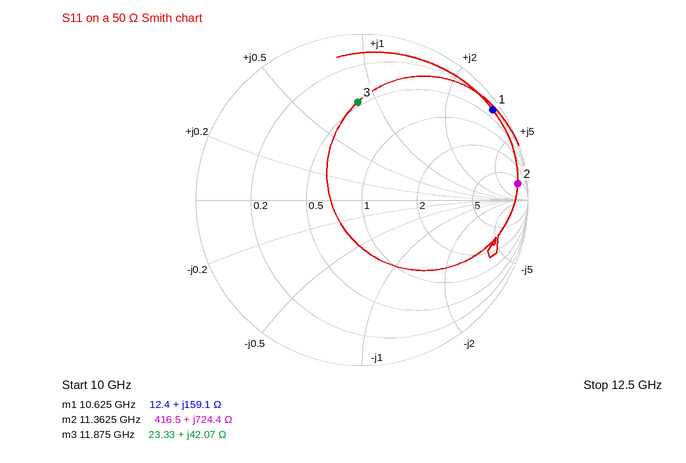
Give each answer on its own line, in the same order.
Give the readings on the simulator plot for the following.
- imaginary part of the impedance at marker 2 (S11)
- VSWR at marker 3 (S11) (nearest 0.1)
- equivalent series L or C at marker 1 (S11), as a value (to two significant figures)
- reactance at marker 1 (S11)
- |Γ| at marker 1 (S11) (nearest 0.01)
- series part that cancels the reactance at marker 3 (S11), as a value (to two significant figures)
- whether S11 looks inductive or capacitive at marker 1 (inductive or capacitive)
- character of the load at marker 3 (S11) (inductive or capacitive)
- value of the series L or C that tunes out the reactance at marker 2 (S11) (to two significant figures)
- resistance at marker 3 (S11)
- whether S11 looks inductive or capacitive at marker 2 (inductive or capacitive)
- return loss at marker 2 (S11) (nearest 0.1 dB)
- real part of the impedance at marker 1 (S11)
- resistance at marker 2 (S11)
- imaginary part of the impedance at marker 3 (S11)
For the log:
+724.4 Ω
3.9
2.4 nH
+159.1 Ω
0.96
320 fF
inductive
inductive
19 fF
23.33 Ω
inductive
0.5 dB
12.4 Ω
416.5 Ω
+42.07 Ω
